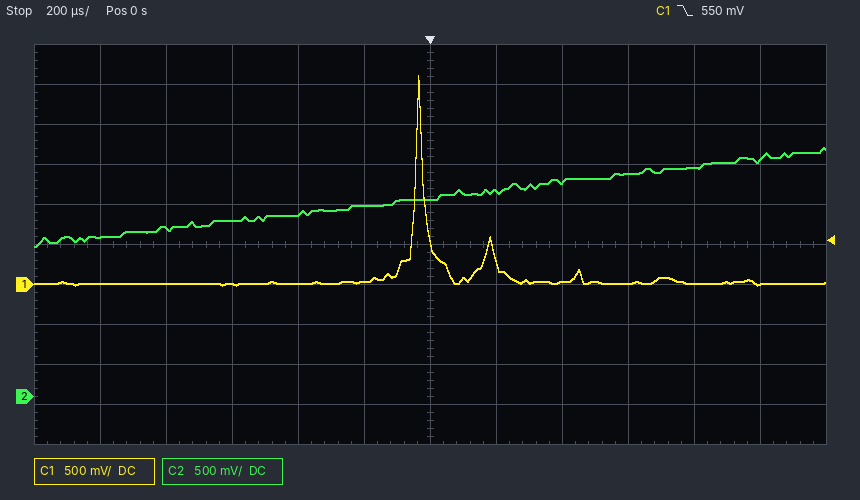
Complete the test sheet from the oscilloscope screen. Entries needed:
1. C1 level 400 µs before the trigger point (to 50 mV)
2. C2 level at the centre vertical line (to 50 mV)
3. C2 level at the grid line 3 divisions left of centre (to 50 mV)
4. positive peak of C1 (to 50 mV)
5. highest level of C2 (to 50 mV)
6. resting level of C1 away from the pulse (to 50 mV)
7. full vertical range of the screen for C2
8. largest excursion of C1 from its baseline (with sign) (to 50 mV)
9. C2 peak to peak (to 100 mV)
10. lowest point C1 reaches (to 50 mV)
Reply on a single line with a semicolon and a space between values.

0 mV; 2.45 V; 2.20 V; 2.60 V; 3.10 V; 0 mV; 5 V; +2.60 V; 1.20 V; 0 mV
